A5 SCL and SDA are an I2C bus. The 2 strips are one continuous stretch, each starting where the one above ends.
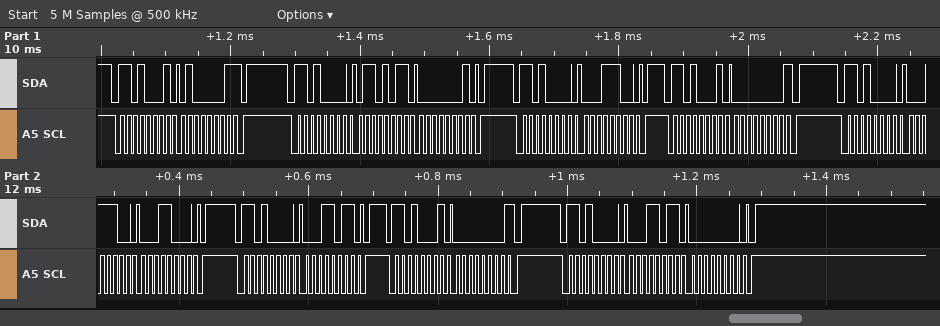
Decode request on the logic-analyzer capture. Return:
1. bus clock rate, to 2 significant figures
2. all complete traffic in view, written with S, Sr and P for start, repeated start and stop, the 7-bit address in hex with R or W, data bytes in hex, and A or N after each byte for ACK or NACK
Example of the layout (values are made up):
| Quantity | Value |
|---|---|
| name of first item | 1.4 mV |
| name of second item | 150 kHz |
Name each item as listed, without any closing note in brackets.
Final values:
| Quantity | Value |
|---|---|
| bus clock rate, to 2 significant figures | 100 kHz |
| all complete traffic in view, written with S, Sr and P for start, repeated start and stop, the 7-bit address in hex with R or W, data bytes in hex, and A or N after each byte for ACK or NACK | S 68R A 41 N P S 68W A 6B A 01 A P S 68W A 1C A P S 68R A 00 N P S 68W A 1C A 18 A P S 68W A 1B A P S 68R A 00 N P S 68W A 1B A 00 A P |
